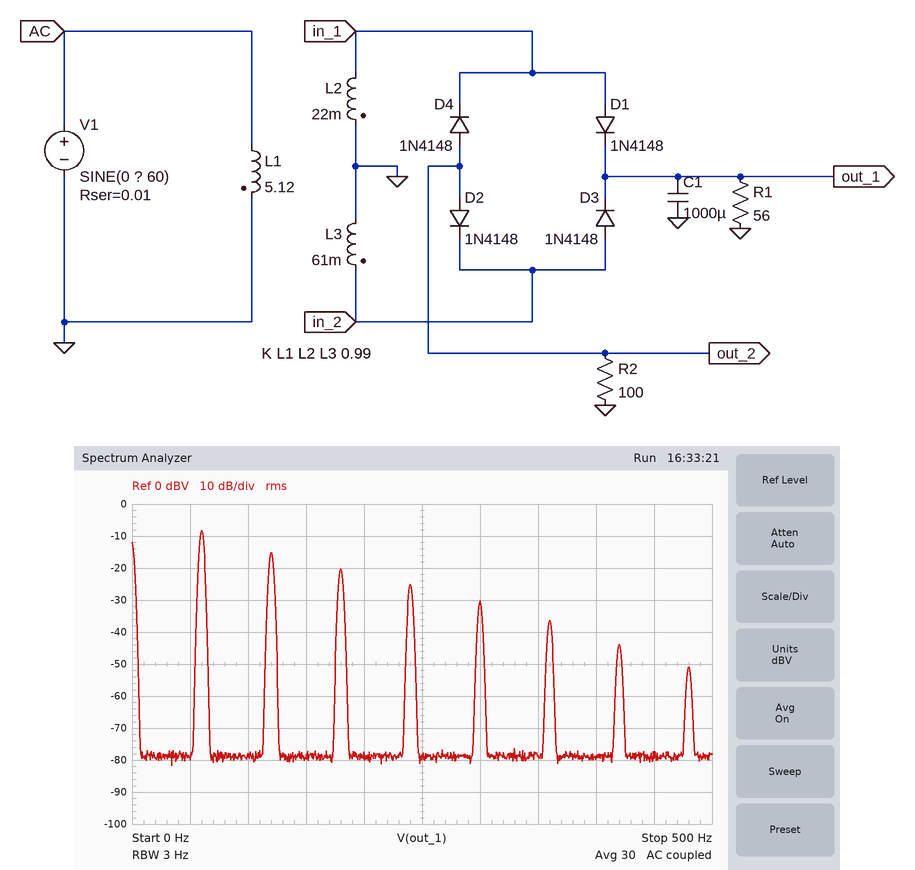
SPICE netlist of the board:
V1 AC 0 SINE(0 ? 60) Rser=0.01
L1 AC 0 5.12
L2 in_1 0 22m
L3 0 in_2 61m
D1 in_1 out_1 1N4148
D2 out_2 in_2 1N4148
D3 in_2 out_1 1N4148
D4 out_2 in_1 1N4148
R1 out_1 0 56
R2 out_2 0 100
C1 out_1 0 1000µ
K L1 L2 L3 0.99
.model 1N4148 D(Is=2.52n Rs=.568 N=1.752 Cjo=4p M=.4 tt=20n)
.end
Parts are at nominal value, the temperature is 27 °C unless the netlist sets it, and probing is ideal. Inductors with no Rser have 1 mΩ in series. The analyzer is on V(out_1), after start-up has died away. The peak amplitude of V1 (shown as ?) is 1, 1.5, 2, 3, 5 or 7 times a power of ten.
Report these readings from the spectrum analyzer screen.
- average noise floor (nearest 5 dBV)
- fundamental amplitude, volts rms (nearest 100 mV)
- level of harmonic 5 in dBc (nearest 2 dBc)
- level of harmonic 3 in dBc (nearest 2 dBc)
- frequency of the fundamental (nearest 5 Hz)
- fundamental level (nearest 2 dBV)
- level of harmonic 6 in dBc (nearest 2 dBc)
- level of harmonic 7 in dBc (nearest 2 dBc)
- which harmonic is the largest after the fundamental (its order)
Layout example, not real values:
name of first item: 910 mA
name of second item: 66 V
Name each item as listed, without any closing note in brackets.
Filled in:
average noise floor: -80 dBV
fundamental amplitude, volts rms: 400 mV
level of harmonic 5 in dBc: -22 dBc
level of harmonic 3 in dBc: -12 dBc
frequency of the fundamental: 60 Hz
fundamental level: -8 dBV
level of harmonic 6 in dBc: -28 dBc
level of harmonic 7 in dBc: -36 dBc
which harmonic is the largest after the fundamental: 2
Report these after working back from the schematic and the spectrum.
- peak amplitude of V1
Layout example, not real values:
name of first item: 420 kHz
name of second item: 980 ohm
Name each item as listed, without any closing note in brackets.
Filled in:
peak amplitude of V1: 70 V
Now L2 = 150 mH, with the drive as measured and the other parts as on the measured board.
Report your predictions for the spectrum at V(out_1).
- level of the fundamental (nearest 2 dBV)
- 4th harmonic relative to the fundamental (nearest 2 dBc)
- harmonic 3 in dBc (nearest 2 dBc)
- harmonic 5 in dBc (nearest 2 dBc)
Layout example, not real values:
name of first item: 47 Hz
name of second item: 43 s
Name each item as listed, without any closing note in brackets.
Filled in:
level of the fundamental: -4 dBV
4th harmonic relative to the fundamental: -20 dBc
harmonic 3 in dBc: -14 dBc
harmonic 5 in dBc: -28 dBc
